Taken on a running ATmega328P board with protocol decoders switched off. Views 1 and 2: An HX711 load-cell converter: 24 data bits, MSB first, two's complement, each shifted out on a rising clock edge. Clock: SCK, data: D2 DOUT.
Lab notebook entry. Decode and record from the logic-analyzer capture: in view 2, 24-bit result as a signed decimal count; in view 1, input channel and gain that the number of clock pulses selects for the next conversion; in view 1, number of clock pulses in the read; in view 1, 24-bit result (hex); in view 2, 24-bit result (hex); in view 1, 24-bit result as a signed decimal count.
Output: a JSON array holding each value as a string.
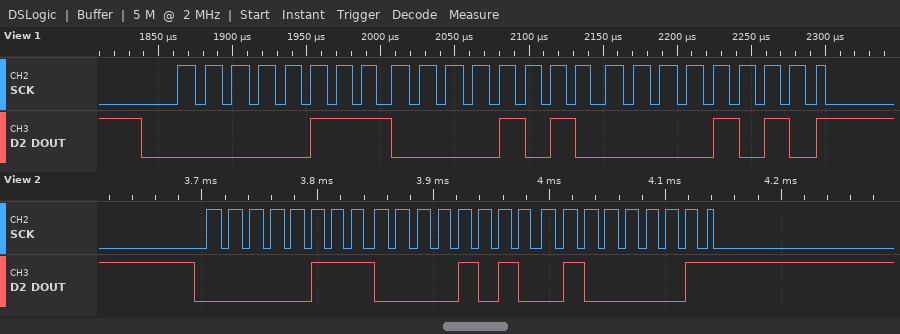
["461377", "channel A, gain 128", "25", "0x070A0A", "0x070A41", "461322"]
